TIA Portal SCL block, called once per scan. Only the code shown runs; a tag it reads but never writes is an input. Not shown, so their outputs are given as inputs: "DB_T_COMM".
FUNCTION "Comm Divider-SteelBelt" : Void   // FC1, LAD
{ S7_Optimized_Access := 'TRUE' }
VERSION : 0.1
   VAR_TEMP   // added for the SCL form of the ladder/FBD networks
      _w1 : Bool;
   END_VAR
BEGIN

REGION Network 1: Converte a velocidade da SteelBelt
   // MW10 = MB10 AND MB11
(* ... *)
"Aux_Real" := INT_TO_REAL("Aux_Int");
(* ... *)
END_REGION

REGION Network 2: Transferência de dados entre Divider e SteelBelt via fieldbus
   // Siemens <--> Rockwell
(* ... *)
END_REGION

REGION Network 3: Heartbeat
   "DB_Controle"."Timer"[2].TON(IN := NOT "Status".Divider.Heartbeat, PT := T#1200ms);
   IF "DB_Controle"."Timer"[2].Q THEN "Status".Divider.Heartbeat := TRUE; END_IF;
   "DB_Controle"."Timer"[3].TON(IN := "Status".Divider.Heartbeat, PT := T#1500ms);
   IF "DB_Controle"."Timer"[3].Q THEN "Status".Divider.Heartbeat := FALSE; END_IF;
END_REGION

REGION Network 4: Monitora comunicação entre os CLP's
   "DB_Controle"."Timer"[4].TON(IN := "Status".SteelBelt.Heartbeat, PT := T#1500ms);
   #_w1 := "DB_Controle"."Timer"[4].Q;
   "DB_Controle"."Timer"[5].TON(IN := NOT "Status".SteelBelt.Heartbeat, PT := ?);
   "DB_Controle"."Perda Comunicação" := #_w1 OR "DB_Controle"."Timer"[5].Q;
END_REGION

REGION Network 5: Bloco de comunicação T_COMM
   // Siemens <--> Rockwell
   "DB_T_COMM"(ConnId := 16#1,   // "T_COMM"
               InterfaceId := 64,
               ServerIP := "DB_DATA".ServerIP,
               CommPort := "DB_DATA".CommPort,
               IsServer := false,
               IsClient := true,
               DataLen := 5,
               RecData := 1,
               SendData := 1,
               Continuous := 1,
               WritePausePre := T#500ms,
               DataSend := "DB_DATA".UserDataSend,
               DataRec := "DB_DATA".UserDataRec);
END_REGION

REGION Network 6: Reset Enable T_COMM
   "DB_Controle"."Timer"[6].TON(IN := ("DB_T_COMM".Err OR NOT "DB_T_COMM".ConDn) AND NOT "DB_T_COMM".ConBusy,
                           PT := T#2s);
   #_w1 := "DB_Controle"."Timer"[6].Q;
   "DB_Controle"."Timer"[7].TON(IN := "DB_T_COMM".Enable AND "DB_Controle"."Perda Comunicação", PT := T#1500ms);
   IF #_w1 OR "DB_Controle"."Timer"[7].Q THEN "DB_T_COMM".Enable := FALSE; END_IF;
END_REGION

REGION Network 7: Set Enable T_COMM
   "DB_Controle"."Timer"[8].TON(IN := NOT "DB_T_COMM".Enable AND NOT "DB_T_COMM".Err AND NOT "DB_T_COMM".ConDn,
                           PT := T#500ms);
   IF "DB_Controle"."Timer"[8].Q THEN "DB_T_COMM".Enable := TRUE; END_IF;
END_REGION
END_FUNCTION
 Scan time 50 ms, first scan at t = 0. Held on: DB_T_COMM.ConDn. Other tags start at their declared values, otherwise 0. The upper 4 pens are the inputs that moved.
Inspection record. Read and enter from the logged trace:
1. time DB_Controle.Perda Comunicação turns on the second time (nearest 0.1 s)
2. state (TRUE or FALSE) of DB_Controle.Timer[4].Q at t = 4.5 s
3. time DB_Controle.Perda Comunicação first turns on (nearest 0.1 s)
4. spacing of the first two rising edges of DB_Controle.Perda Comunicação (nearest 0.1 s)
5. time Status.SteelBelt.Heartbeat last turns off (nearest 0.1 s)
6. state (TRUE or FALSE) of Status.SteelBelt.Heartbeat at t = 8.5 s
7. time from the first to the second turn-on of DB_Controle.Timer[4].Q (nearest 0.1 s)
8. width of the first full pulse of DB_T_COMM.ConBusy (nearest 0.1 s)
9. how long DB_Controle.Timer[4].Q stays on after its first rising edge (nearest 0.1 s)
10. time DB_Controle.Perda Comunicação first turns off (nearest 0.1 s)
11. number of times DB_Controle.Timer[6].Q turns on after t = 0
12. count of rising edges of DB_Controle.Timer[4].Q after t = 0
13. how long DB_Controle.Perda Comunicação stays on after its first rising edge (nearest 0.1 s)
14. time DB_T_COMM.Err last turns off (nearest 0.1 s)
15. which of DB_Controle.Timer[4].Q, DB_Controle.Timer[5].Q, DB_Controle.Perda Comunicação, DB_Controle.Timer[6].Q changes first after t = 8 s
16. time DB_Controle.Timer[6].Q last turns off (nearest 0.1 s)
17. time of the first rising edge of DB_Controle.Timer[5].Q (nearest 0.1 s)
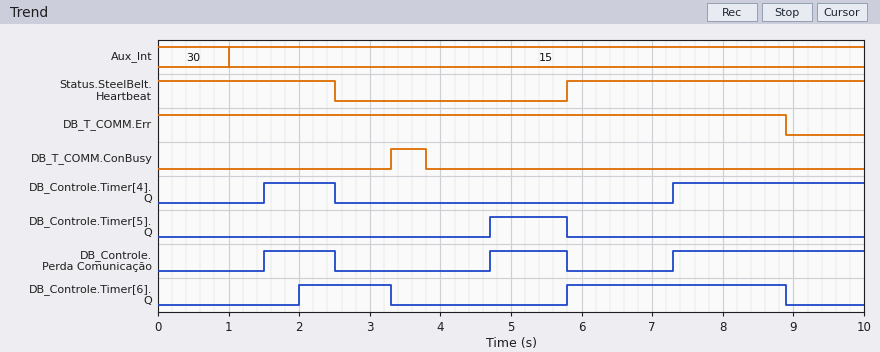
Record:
4.7 s
FALSE
1.5 s
3.2 s
2.5 s
TRUE
5.8 s
0.5 s
1.0 s
2.5 s
2
2
1.0 s
8.9 s
DB_Controle.Timer[6].Q
8.9 s
4.7 s
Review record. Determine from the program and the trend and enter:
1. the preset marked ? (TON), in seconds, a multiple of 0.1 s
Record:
2.2 s
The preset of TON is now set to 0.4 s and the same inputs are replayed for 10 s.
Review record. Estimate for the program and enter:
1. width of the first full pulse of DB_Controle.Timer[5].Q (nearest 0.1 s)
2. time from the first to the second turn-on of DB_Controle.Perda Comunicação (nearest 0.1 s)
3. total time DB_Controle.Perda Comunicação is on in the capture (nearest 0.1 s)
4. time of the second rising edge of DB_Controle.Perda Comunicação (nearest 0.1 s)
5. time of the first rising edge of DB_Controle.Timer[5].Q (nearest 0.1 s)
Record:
2.9 s
1.4 s
6.6 s
2.9 s
2.9 s
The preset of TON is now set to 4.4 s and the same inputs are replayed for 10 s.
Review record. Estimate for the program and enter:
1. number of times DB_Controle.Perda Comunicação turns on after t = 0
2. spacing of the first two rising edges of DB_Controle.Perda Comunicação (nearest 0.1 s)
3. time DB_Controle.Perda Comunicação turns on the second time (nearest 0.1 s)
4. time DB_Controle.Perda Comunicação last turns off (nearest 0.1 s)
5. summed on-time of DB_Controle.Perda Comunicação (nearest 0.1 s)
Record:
2
5.8 s
7.3 s
2.5 s
3.7 s
